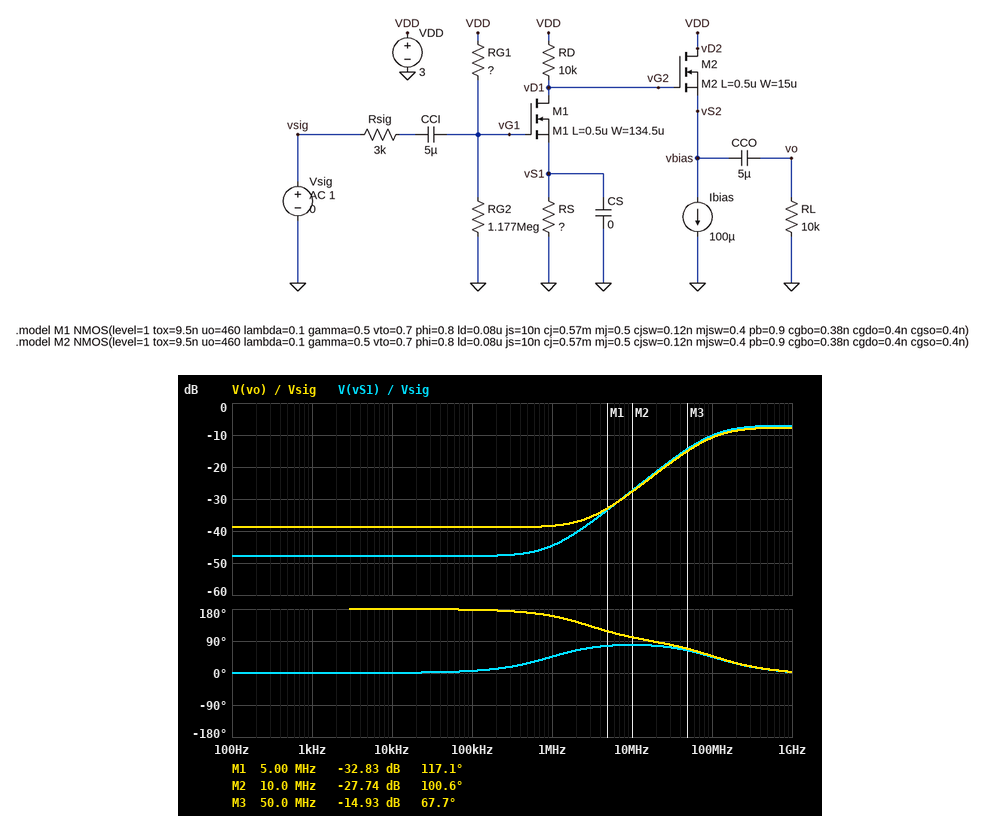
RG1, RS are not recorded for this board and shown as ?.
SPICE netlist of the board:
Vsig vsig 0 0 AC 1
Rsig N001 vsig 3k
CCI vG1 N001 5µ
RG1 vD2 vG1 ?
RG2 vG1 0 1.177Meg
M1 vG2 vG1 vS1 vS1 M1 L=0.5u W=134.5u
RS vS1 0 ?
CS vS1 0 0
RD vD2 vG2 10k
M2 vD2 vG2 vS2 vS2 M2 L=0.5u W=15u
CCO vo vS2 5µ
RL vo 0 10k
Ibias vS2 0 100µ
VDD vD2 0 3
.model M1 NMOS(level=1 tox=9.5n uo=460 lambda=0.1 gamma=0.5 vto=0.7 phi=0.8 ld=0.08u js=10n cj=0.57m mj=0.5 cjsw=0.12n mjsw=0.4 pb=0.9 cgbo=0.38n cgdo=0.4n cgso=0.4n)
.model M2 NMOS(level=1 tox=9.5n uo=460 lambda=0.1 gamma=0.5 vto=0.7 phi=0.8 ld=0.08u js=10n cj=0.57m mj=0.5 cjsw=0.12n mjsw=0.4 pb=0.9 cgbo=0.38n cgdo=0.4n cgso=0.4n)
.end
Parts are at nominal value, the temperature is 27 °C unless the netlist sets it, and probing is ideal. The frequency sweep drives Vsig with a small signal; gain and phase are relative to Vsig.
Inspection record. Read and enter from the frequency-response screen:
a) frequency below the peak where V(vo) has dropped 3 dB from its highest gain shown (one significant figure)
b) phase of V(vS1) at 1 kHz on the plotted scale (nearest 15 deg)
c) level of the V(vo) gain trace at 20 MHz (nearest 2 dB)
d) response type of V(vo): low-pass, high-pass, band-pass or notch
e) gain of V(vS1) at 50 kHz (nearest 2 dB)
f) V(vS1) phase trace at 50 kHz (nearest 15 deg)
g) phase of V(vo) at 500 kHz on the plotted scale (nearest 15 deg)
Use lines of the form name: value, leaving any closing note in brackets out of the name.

frequency below the peak where V(vo) has dropped 3 dB from its highest gain shown: 100 MHz
phase of V(vS1) at 1 kHz on the plotted scale: 0 deg
level of the V(vo) gain trace at 20 MHz: -22 dB
response type of V(vo): low-pass, high-pass, band-pass or notch: high-pass
gain of V(vS1) at 50 kHz: -48 dB
V(vS1) phase trace at 50 kHz: 0 deg
phase of V(vo) at 500 kHz on the plotted scale: 165 deg
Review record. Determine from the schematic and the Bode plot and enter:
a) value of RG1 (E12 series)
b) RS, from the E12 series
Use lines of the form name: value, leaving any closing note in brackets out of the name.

value of RG1: 680 kΩ
RS, from the E12 series: 3.3 kΩ
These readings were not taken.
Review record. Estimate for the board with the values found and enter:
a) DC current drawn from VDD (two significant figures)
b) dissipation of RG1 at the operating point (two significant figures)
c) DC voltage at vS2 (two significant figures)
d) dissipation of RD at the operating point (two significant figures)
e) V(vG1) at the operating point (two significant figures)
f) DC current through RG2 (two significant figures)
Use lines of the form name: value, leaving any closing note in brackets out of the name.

DC current drawn from VDD: 330 µA
dissipation of RG1 at the operating point: 1.8 µW
DC voltage at vS2: -94 mV
dissipation of RD at the operating point: 510 µW
V(vG1) at the operating point: 1.9 V
DC current through RG2: 1.6 µA
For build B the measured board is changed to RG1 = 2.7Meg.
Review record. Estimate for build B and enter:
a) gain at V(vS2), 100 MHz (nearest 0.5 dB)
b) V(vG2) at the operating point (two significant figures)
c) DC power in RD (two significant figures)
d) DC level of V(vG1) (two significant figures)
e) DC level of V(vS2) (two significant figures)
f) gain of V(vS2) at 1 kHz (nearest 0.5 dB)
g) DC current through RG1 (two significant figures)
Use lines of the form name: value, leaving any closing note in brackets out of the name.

gain at V(vS2), 100 MHz: 6.0 dB
V(vG2) at the operating point: 2.5 V
DC power in RD: 28 µW
DC level of V(vG1): 910 mV
DC level of V(vS2): 1.6 V
gain of V(vS2) at 1 kHz: 8.0 dB
DC current through RG1: 770 nA
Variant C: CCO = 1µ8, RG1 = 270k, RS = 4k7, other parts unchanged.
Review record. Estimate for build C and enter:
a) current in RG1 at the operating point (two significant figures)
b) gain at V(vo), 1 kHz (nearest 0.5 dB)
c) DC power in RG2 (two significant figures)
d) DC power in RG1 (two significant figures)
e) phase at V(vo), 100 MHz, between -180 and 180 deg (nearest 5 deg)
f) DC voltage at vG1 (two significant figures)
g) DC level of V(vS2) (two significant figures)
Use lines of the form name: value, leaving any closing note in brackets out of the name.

current in RG1 at the operating point: 2.1 µA
gain at V(vo), 1 kHz: -50.0 dB
DC power in RG2: 5.1 µW
DC power in RG1: 1.2 µW
phase at V(vo), 100 MHz, between -180 and 180 deg: 45 deg
DC voltage at vG1: 2.4 V
DC level of V(vS2): 120 mV
